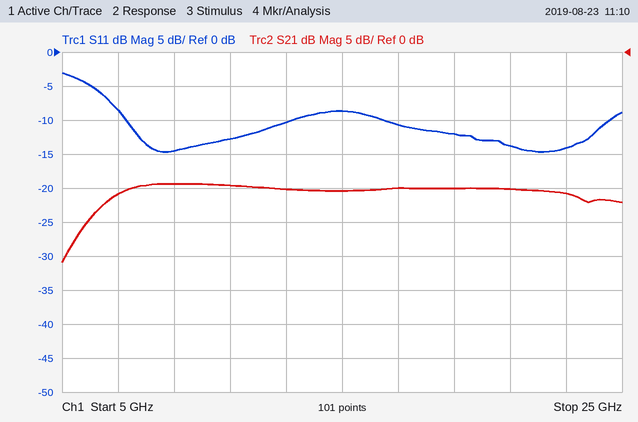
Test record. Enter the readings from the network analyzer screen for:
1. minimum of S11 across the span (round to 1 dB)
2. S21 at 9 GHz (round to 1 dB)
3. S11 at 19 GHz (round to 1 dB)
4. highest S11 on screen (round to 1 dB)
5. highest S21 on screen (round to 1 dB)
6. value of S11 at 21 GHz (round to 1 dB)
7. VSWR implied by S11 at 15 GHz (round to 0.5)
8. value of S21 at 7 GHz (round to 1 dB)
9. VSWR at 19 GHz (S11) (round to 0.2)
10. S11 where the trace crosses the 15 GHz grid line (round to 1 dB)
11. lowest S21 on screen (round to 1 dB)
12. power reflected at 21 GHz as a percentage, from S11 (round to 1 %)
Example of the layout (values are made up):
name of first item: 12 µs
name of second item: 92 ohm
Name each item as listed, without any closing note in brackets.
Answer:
minimum of S11 across the span: -15 dB
S21 at 9 GHz: -19 dB
S11 at 19 GHz: -12 dB
highest S11 on screen: -3 dB
highest S21 on screen: -19 dB
value of S11 at 21 GHz: -14 dB
VSWR implied by S11 at 15 GHz: 2.0
value of S21 at 7 GHz: -21 dB
VSWR at 19 GHz (S11): 1.6
S11 where the trace crosses the 15 GHz grid line: -9 dB
lowest S21 on screen: -31 dB
power reflected at 21 GHz as a percentage, from S11: 4 %
